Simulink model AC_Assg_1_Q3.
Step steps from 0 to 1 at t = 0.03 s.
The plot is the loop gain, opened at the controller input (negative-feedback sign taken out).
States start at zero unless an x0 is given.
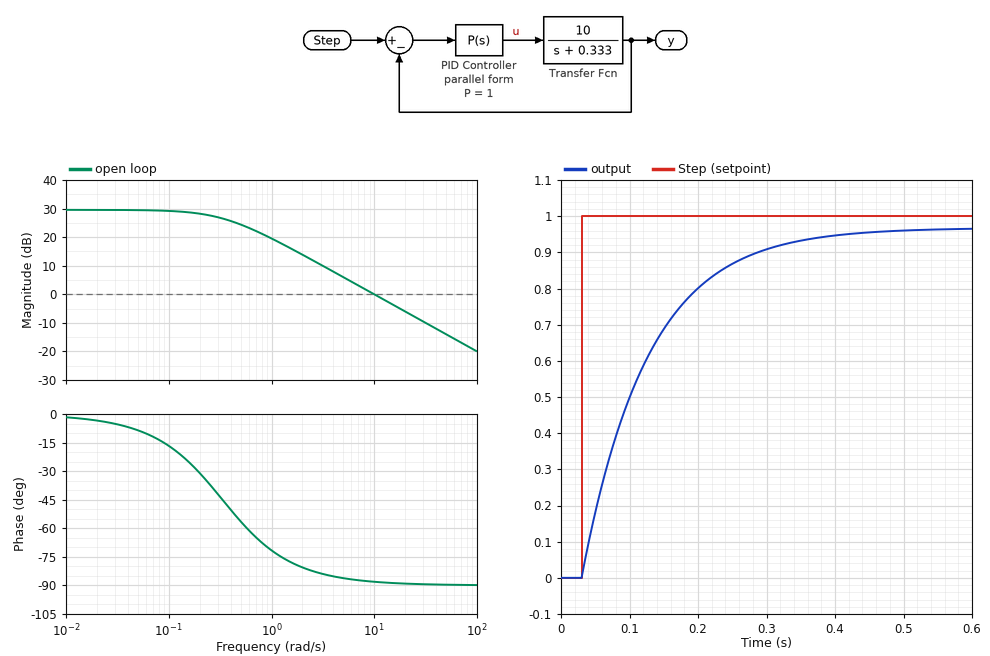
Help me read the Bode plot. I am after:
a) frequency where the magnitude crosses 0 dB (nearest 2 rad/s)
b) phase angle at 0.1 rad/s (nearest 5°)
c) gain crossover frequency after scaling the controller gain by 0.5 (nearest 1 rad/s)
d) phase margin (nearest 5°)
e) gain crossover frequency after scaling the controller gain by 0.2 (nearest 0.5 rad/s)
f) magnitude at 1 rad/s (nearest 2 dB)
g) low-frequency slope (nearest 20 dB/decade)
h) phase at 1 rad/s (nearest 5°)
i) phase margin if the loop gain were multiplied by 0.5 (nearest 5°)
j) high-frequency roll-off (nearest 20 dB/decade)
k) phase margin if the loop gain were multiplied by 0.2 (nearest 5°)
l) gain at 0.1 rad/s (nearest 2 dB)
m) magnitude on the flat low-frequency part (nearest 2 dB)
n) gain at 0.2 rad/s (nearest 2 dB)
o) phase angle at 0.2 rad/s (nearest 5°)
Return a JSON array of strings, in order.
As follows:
["10 rad/s", "-15°", "5 rad/s", "90°", "2.0 rad/s", "20 dB", "0 dB/decade", "-70°", "95°", "-20 dB/decade", "100°", "30 dB", "30 dB", "28 dB", "-30°"]
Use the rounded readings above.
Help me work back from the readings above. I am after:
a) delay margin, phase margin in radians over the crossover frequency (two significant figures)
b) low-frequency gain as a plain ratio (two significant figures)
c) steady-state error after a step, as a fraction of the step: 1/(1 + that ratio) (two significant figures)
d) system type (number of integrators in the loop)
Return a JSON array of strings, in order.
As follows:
["0.16 s", "32", "0.030", "0"]
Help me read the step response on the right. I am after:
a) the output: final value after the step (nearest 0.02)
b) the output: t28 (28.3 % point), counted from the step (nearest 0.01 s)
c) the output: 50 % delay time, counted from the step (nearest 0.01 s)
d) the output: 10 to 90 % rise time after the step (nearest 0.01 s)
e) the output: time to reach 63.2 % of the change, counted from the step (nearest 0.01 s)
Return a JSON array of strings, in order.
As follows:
["0.96", "0.03 s", "0.07 s", "0.21 s", "0.10 s"]
